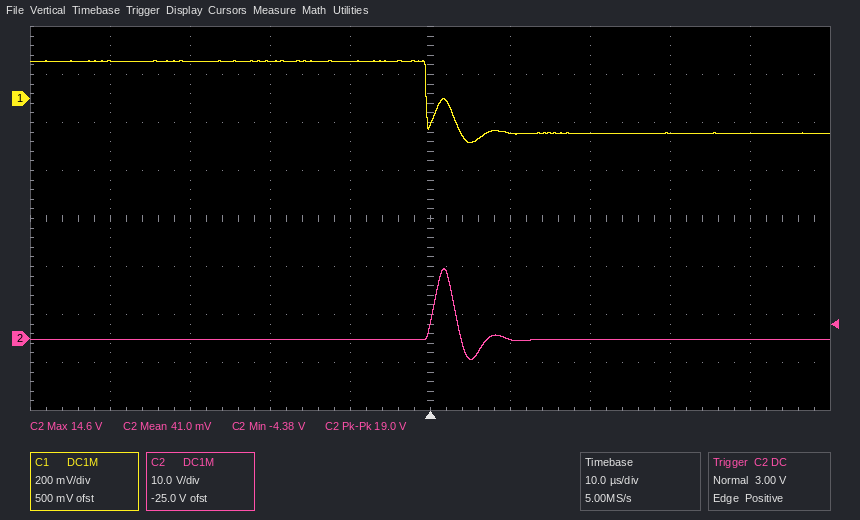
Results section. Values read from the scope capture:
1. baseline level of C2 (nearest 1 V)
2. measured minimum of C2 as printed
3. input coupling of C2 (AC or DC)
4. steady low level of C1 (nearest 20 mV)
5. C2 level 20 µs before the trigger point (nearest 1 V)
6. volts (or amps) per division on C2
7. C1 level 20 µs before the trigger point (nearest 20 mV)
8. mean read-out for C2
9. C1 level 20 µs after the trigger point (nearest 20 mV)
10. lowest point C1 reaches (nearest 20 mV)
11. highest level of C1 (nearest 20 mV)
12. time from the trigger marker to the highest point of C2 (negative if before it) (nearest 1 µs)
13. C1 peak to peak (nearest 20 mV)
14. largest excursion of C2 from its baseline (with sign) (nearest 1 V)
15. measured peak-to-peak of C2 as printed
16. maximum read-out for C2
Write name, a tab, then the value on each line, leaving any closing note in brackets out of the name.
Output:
baseline level of C2	0 V
measured minimum of C2 as printed	-4.38 V
input coupling of C2	DC
steady low level of C1	-140 mV
C2 level 20 µs before the trigger point	0 V
volts (or amps) per division on C2	10 V
C1 level 20 µs before the trigger point	160 mV
mean read-out for C2	41.0 mV
C1 level 20 µs after the trigger point	-140 mV
lowest point C1 reaches	-180 mV
highest level of C1	160 mV
time from the trigger marker to the highest point of C2 (negative if before it)	+2 µs
C1 peak to peak	340 mV
largest excursion of C2 from its baseline (with sign)	+15 V
measured peak-to-peak of C2 as printed	19.0 V
maximum read-out for C2	14.6 V
